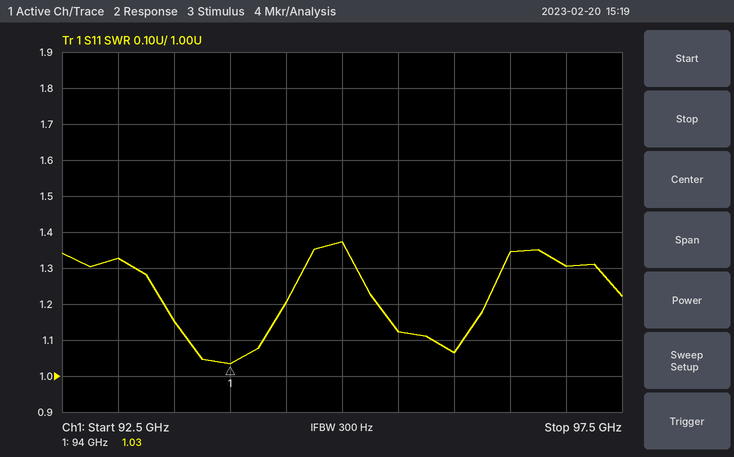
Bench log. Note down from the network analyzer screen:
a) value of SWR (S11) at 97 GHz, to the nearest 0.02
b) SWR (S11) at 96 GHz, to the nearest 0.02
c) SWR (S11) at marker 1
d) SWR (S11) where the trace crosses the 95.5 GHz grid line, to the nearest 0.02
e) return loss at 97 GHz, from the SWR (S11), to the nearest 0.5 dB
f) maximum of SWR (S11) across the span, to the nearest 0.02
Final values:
1.30
1.06
1.03
1.12
17.5 dB
1.38
